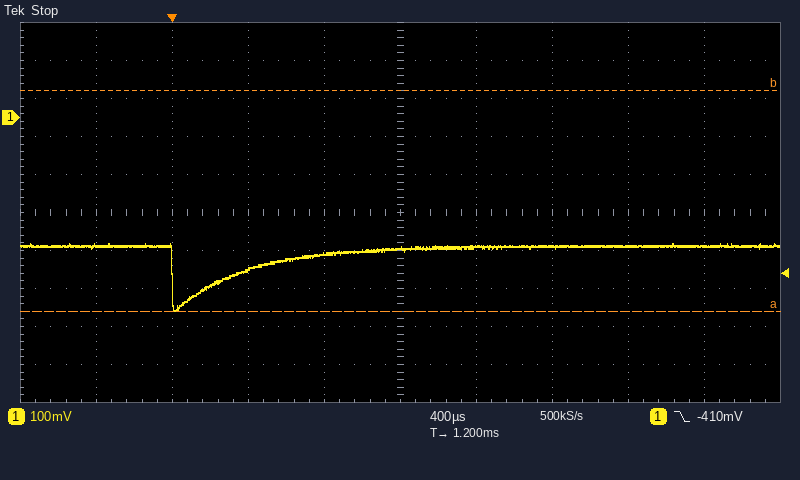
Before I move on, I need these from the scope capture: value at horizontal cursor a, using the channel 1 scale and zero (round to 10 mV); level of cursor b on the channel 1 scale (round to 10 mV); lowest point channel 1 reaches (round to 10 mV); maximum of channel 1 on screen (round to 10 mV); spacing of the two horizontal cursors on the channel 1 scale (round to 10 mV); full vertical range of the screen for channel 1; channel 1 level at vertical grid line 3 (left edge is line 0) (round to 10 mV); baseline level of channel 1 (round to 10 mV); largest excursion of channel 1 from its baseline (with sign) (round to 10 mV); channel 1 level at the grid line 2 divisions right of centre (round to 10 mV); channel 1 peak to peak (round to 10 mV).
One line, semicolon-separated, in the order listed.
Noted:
-510 mV; 70 mV; -510 mV; -330 mV; 580 mV; 1 V; -400 mV; -340 mV; -170 mV; -340 mV; 180 mV
